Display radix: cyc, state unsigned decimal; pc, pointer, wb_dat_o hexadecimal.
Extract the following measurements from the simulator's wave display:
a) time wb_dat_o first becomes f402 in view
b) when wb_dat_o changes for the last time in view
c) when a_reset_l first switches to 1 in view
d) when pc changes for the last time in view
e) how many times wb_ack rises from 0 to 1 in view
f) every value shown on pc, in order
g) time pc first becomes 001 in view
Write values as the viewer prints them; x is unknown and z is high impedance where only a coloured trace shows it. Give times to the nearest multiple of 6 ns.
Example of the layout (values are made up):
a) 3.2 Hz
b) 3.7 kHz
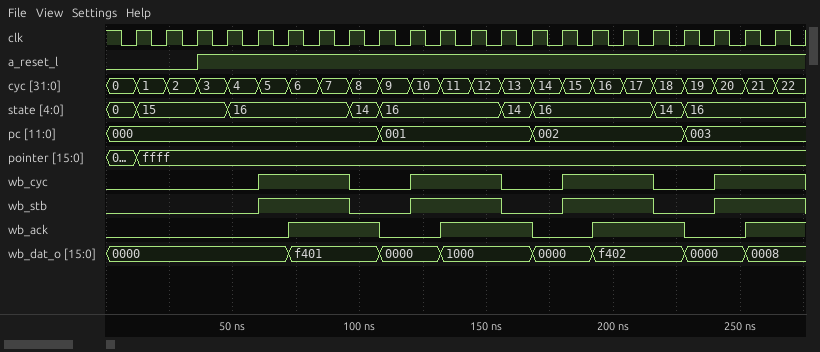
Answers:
a) 192 ns
b) 252 ns
c) 36 ns
d) 228 ns
e) 4
f) 000, 001, 002, 003
g) 108 ns
